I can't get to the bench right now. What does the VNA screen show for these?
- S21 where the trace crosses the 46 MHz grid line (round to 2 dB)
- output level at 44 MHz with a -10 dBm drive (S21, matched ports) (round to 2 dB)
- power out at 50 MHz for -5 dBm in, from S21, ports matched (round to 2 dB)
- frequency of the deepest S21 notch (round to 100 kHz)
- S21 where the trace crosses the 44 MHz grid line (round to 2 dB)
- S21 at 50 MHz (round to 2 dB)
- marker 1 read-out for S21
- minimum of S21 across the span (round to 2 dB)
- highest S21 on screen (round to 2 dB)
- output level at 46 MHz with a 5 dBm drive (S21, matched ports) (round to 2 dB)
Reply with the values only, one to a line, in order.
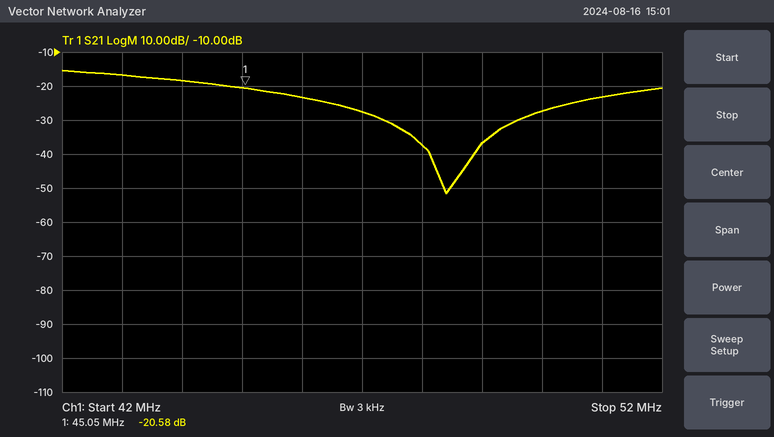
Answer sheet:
-24 dB
-28 dBm
-32 dBm
48.4 MHz
-18 dB
-28 dB
-20.58 dB
-52 dB
-16 dB
-18 dBm
